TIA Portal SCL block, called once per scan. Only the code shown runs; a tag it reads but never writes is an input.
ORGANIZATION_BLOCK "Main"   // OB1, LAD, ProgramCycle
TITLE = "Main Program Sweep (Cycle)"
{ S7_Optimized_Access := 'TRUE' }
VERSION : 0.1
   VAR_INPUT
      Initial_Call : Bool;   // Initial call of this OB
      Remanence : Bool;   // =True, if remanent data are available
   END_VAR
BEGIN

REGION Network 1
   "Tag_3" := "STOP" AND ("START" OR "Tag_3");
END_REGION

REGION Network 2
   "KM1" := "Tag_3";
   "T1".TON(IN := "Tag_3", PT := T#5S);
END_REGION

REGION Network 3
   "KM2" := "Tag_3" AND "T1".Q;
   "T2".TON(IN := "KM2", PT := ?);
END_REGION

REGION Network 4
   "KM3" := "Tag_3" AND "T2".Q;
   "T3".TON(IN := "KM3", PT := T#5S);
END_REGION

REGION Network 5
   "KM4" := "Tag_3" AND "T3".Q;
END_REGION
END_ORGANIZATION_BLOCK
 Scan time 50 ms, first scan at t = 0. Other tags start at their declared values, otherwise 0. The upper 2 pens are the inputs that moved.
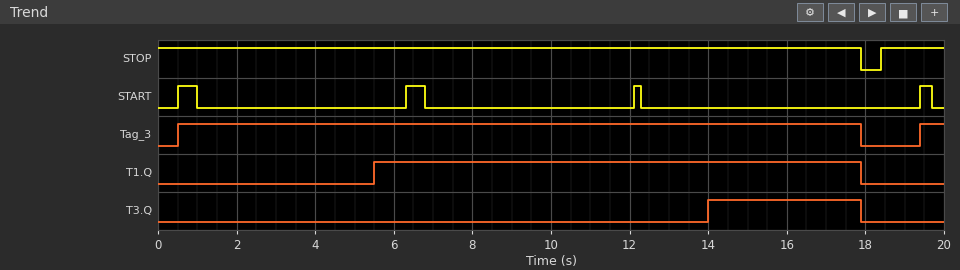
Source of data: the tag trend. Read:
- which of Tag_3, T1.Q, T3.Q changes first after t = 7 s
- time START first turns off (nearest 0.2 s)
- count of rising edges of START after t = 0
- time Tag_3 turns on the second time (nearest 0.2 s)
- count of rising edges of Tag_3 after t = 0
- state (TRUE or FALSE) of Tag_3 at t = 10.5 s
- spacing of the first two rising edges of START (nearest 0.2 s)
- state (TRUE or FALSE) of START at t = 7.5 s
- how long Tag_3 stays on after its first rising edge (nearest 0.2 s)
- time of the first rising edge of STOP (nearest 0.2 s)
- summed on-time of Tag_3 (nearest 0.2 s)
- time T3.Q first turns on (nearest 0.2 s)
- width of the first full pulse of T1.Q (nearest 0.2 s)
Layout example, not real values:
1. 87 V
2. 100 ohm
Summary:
1. T3.Q
2. 1.0 s
3. 4
4. 19.4 s
5. 2
6. TRUE
7. 5.8 s
8. FALSE
9. 17.4 s
10. 18.4 s
11. 18.0 s
12. 14.0 s
13. 12.4 s
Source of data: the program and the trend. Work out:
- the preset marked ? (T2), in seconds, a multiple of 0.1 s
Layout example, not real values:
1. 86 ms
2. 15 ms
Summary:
1. 3.5 s
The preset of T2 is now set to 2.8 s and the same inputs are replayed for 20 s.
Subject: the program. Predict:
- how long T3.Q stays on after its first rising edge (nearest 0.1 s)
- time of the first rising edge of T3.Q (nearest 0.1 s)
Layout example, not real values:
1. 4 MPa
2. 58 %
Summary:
1. 4.6 s
2. 13.3 s
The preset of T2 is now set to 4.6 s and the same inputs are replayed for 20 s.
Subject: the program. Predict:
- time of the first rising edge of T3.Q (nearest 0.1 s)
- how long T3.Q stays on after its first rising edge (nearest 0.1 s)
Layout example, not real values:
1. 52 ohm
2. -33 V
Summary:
1. 15.1 s
2. 2.8 s
